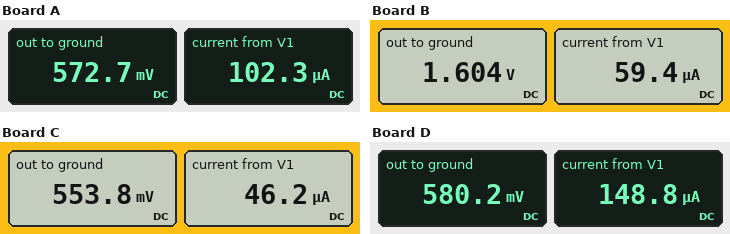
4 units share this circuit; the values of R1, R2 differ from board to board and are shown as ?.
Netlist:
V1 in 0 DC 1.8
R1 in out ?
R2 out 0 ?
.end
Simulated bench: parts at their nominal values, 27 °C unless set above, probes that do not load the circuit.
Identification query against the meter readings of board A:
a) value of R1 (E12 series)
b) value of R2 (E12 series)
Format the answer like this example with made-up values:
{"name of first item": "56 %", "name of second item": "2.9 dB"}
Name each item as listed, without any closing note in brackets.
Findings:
{"value of R1": "12 kΩ", "value of R2": "5.6 kΩ"}
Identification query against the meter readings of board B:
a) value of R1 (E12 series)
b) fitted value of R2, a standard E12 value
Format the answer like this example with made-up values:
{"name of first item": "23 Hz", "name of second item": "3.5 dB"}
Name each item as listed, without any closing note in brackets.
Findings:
{"value of R1": "3.3 kΩ", "fitted value of R2, a standard E12 value": "27 kΩ"}
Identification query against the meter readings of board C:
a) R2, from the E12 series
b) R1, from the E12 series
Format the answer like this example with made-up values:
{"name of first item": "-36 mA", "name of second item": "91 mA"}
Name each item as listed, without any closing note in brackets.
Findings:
{"R2, from the E12 series": "12 kΩ", "R1, from the E12 series": "27 kΩ"}
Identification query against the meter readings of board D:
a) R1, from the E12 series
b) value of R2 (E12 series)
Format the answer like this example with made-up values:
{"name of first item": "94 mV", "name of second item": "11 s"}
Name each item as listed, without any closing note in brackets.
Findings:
{"R1, from the E12 series": "8.2 kΩ", "value of R2": "3.9 kΩ"}
